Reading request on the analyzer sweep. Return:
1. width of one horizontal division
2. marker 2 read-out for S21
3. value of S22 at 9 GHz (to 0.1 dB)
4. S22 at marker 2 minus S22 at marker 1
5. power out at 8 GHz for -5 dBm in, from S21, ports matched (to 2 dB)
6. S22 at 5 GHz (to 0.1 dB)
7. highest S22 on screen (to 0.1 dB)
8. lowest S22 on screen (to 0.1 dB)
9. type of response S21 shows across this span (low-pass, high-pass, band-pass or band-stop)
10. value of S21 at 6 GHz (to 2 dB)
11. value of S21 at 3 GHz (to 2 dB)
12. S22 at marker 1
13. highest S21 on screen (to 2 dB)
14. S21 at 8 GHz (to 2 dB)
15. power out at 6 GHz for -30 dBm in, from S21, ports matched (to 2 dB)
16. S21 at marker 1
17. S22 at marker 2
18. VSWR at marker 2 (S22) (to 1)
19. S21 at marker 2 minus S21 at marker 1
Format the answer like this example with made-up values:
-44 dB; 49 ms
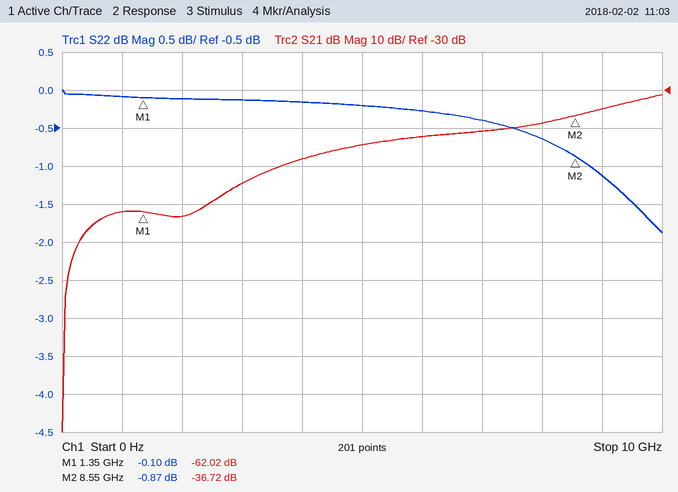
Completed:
1 GHz; -36.72 dB; -1.1 dB; -0.77 dB; -44 dBm; -0.2 dB; 0.0 dB; -1.9 dB; high-pass; -42 dB; -54 dB; -0.10 dB; -32 dB; -38 dB; -72 dBm; -62.02 dB; -0.87 dB; 20; 25.30 dB
